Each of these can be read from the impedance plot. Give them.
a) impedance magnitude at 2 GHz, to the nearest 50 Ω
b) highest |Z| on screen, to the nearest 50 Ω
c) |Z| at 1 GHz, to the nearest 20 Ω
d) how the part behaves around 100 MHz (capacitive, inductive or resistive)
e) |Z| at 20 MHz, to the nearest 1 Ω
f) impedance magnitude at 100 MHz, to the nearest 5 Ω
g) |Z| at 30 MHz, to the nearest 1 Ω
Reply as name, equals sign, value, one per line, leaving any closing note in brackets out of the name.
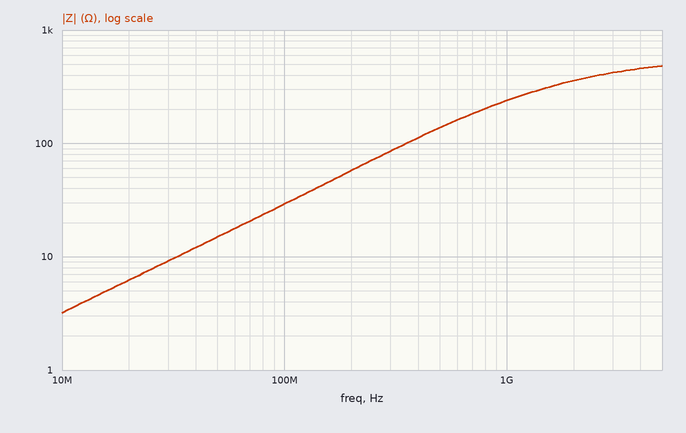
impedance magnitude at 2 GHz, to the nearest 50 Ω = 350 Ω
highest |Z| on screen, to the nearest 50 Ω = 500 Ω
|Z| at 1 GHz, to the nearest 20 Ω = 240 Ω
how the part behaves around 100 MHz = inductive
|Z| at 20 MHz, to the nearest 1 Ω = 6 Ω
impedance magnitude at 100 MHz, to the nearest 5 Ω = 30 Ω
|Z| at 30 MHz, to the nearest 1 Ω = 9 Ω
